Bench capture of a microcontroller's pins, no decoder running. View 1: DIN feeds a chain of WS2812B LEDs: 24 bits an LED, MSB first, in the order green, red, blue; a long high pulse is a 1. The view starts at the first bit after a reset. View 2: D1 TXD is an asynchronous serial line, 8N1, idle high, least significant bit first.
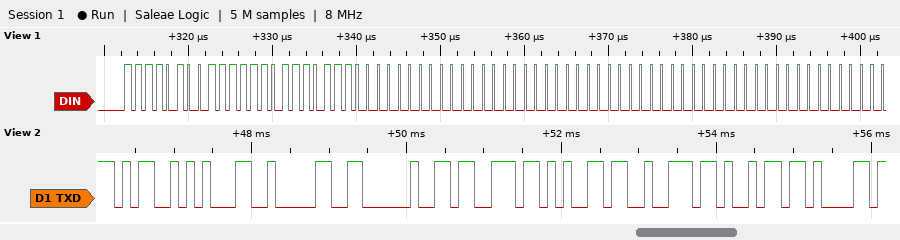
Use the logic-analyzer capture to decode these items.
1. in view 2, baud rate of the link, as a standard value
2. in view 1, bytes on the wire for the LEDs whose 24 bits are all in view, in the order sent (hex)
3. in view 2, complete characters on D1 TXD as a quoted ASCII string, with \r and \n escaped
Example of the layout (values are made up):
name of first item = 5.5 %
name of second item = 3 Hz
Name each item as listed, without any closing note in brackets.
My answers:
in view 2, baud rate of the link, as a standard value = 9600 baud
in view 1, bytes on the wire for the LEDs whose 24 bits are all in view, in the order sent = F4 FD DC 00 00 00 00 00 00
in view 2, complete characters on D1 TXD as a quoted ASCII string, with \r and \n escaped = "M10 seria"
